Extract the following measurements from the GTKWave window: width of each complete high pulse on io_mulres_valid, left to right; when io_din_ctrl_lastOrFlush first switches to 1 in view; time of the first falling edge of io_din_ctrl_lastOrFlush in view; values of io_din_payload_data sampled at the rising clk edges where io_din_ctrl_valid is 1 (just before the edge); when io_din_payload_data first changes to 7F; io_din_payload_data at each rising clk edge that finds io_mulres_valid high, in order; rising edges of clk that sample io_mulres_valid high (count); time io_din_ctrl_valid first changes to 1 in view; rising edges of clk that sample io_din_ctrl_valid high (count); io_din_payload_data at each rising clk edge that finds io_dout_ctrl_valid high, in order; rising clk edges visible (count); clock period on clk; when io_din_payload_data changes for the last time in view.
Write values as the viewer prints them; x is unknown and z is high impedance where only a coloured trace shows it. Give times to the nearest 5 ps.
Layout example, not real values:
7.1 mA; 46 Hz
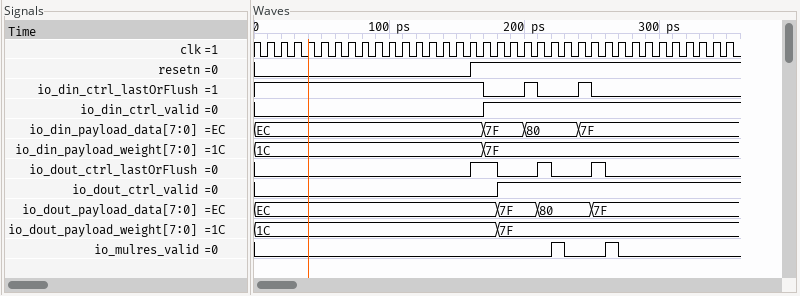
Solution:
10 ps, 10 ps; 200 ps; 170 ps; 7F, 7F, 7F, 80, 80, 80, 80, 7F, 7F, 7F, 7F, 7F, 7F, 7F, 7F, 7F, 7F, 7F; 170 ps; 80, 7F; 2; 170 ps; 18; 7F, 7F, 80, 80, 80, 80, 7F, 7F, 7F, 7F, 7F, 7F, 7F, 7F, 7F, 7F, 7F; 35; 10 ps; 240 ps
